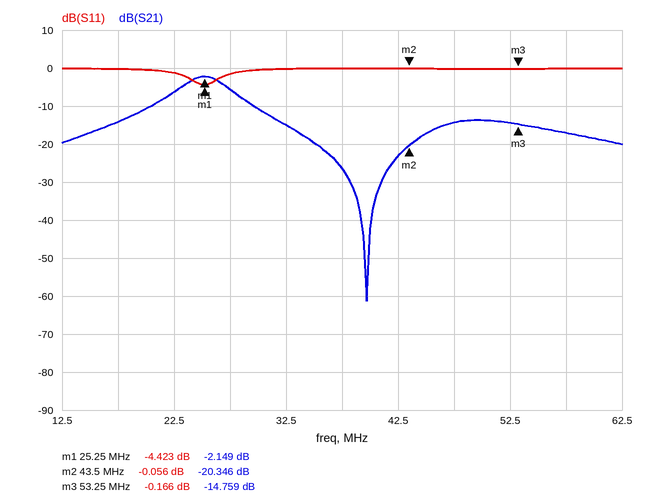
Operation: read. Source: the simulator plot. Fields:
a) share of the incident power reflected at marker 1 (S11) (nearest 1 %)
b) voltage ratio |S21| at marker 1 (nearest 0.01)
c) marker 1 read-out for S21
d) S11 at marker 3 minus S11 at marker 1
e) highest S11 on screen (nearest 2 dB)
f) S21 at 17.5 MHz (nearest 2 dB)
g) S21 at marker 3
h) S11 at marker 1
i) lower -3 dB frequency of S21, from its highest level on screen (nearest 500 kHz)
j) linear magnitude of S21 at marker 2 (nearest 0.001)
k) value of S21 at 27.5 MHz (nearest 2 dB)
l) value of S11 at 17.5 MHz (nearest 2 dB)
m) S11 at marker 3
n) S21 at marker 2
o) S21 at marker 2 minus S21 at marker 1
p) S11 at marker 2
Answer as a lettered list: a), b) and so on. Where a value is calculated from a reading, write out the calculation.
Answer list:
a) 10^(-4.423/10) ≈ 36 %
b) 10^(-2.149/20) ≈ 0.78
c) -2.149 dB
d) -0.166 − (-4.423) = 4.257 dB
e) 0 dB
f) -14 dB
g) -14.759 dB
h) -4.423 dB
i) 23.0 MHz
j) 10^(-20.346/20) ≈ 0.096
k) -6 dB
l) 0 dB
m) -0.166 dB
n) -20.346 dB
o) -20.346 − (-2.149) = -18.197 dB
p) -0.056 dB
